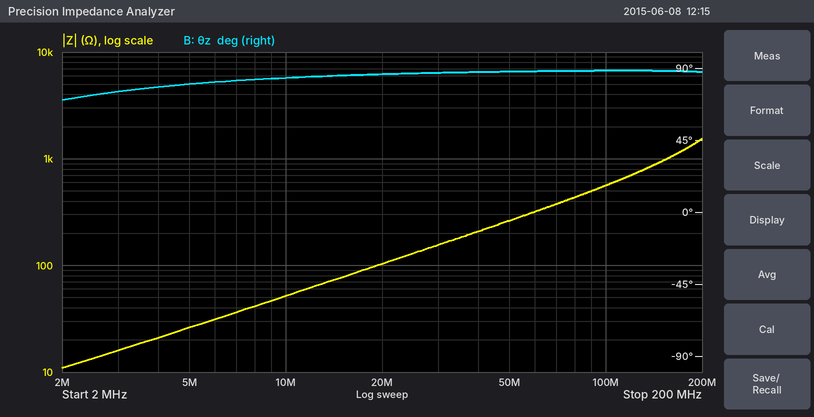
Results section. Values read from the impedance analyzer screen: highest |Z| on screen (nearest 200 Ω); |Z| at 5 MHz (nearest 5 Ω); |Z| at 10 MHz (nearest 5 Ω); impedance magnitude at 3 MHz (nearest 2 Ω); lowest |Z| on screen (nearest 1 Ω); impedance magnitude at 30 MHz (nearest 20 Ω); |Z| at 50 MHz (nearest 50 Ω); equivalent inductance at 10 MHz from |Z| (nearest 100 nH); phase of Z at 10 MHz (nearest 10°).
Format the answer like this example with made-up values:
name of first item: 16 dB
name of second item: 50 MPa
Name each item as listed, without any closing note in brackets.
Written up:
highest |Z| on screen: 1.6 kΩ
|Z| at 5 MHz: 25 Ω
|Z| at 10 MHz: 50 Ω
impedance magnitude at 3 MHz: 16 Ω
lowest |Z| on screen: 11 Ω
impedance magnitude at 30 MHz: 160 Ω
|Z| at 50 MHz: 250 Ω
equivalent inductance at 10 MHz from |Z|: 800 nH
phase of Z at 10 MHz: 80°
